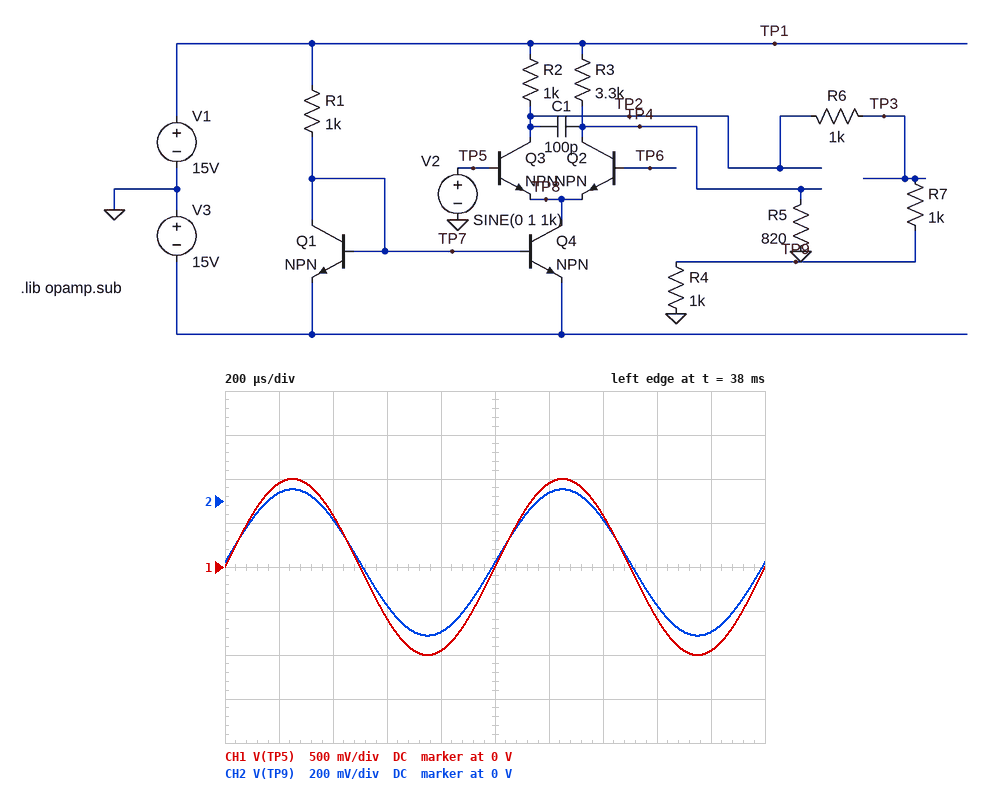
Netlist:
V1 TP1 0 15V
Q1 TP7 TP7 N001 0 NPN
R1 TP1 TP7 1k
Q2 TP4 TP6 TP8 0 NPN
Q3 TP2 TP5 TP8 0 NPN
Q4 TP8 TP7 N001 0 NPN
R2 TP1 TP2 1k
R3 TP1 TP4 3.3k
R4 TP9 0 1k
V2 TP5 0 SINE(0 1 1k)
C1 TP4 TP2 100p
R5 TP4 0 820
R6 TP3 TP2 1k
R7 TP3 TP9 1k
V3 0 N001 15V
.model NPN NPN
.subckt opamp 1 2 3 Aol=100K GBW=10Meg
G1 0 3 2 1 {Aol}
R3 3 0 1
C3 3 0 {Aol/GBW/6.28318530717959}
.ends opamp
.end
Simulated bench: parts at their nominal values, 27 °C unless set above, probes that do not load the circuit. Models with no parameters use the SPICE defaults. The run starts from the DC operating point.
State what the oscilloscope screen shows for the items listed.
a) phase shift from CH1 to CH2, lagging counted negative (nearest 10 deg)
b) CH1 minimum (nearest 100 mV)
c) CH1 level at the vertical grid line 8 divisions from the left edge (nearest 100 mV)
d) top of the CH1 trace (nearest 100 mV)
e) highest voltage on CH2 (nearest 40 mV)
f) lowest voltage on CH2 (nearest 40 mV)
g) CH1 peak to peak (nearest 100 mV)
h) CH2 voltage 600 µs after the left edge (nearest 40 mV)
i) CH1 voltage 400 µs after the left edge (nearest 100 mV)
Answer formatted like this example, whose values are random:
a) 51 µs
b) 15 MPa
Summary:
a) 0 deg
b) -1.0 V
c) -600 mV
d) 1.0 V
e) 40 mV
f) -600 mV
g) 2.0 V
h) -480 mV
i) 600 mV
